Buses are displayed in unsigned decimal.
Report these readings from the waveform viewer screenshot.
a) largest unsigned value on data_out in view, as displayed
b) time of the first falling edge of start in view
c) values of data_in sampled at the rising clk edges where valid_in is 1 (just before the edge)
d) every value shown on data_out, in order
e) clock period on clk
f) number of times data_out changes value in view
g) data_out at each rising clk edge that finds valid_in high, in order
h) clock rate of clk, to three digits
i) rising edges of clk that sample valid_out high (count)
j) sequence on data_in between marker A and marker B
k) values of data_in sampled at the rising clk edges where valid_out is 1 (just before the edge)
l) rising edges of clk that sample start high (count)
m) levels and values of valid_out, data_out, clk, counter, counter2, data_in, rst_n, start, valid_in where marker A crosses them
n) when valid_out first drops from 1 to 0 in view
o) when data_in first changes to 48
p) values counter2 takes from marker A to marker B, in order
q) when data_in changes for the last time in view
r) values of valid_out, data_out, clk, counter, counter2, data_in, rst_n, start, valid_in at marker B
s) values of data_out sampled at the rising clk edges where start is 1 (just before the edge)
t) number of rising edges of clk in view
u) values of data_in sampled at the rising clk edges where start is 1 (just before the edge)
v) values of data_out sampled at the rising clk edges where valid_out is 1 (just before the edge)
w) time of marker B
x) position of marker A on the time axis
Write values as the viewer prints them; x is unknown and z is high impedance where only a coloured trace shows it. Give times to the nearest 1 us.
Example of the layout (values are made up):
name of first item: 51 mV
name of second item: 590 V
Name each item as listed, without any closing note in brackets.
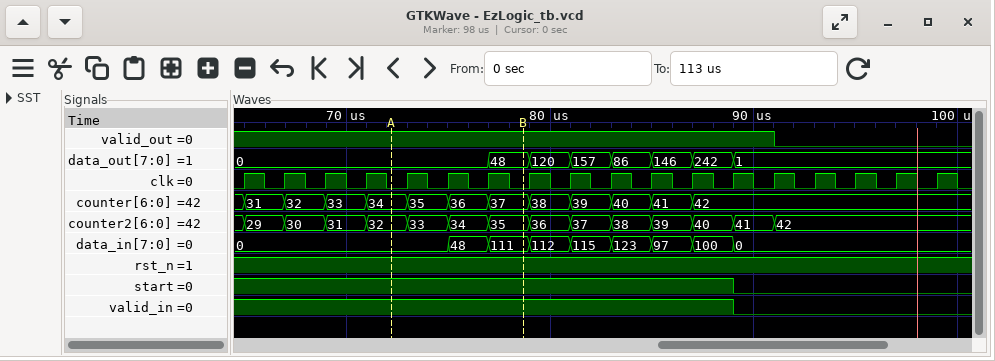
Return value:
largest unsigned value on data_out in view, as displayed: 242
time of the first falling edge of start in view: 89 us
values of data_in sampled at the rising clk edges where valid_in is 1: 0, 0, 0, 0, 0, 0, 48, 111, 112, 115, 123, 97, 100
every value shown on data_out, in order: 0, 48, 120, 157, 86, 146, 242, 1
clock period on clk: 2 us
number of times data_out changes value in view: 7
data_out at each rising clk edge that finds valid_in high, in order: 0, 0, 0, 0, 0, 0, 0, 48, 120, 157, 86, 146, 242
clock rate of clk, to three digits: 500 kHz
rising edges of clk that sample valid_out high: 14
sequence on data_in between marker A and marker B: 0, 48, 111
values of data_in sampled at the rising clk edges where valid_out is 1: 0, 0, 0, 0, 0, 0, 48, 111, 112, 115, 123, 97, 100, 0
rising edges of clk that sample start high: 13
levels and values of valid_out, data_out, clk, counter, counter2, data_in, rst_n, start, valid_in where marker A crosses them: valid_out=1, data_out=0, clk=0, counter=34, counter2=32, data_in=0, rst_n=1, start=1, valid_in=1
when valid_out first drops from 1 to 0 in view: 91 us
when data_in first changes to 48: 75 us
values counter2 takes from marker A to marker B, in order: 32, 33, 34, 35
when data_in changes for the last time in view: 89 us
values of valid_out, data_out, clk, counter, counter2, data_in, rst_n, start, valid_in at marker B: valid_out=1, data_out=48, clk=0, counter=37, counter2=35, data_in=111, rst_n=1, start=1, valid_in=1
values of data_out sampled at the rising clk edges where start is 1: 0, 0, 0, 0, 0, 0, 0, 48, 120, 157, 86, 146, 242
number of rising edges of clk in view: 18
values of data_in sampled at the rising clk edges where start is 1: 0, 0, 0, 0, 0, 0, 48, 111, 112, 115, 123, 97, 100
values of data_out sampled at the rising clk edges where valid_out is 1: 0, 0, 0, 0, 0, 0, 0, 48, 120, 157, 86, 146, 242, 1
time of marker B: 79 us
position of marker A on the time axis: 72 us
